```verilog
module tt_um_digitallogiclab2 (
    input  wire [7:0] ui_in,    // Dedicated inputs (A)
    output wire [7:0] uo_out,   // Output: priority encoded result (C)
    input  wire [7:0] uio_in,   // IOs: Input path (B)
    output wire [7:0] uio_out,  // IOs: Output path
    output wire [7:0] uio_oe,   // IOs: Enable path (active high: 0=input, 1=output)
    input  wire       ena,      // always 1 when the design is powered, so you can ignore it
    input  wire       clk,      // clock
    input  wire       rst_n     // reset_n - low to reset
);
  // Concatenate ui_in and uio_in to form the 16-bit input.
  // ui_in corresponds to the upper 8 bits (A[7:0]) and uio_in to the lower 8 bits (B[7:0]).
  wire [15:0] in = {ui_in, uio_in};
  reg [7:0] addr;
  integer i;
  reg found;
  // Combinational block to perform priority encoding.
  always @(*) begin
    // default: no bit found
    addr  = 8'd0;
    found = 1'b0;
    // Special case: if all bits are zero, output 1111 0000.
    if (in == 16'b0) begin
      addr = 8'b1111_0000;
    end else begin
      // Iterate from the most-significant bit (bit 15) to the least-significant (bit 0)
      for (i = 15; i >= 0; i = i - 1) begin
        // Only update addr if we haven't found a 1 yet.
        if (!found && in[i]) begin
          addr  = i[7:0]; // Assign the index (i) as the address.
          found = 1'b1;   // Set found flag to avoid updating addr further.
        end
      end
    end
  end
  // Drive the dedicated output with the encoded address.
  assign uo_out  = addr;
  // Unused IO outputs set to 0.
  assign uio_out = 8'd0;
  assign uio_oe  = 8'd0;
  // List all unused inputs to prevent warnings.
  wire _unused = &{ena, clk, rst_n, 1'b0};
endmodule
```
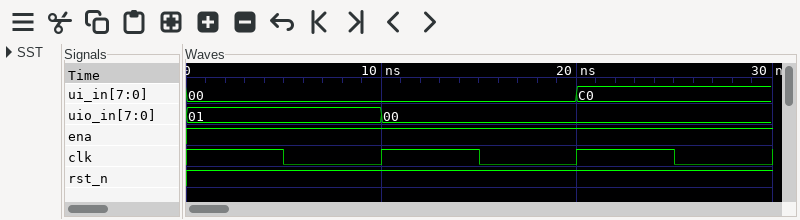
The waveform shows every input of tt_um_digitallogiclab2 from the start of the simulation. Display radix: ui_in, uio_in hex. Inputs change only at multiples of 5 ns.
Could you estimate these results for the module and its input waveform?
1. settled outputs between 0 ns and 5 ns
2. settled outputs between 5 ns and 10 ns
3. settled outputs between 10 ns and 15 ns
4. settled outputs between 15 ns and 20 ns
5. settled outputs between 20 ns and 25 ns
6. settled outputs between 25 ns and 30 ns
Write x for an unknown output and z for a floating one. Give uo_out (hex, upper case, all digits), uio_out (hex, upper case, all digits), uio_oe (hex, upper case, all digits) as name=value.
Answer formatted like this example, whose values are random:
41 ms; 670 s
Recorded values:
uo_out=00, uio_out=00, uio_oe=00; uo_out=00, uio_out=00, uio_oe=00; uo_out=F0, uio_out=00, uio_oe=00; uo_out=F0, uio_out=00, uio_oe=00; uo_out=0F, uio_out=00, uio_oe=00; uo_out=0F, uio_out=00, uio_oe=00
